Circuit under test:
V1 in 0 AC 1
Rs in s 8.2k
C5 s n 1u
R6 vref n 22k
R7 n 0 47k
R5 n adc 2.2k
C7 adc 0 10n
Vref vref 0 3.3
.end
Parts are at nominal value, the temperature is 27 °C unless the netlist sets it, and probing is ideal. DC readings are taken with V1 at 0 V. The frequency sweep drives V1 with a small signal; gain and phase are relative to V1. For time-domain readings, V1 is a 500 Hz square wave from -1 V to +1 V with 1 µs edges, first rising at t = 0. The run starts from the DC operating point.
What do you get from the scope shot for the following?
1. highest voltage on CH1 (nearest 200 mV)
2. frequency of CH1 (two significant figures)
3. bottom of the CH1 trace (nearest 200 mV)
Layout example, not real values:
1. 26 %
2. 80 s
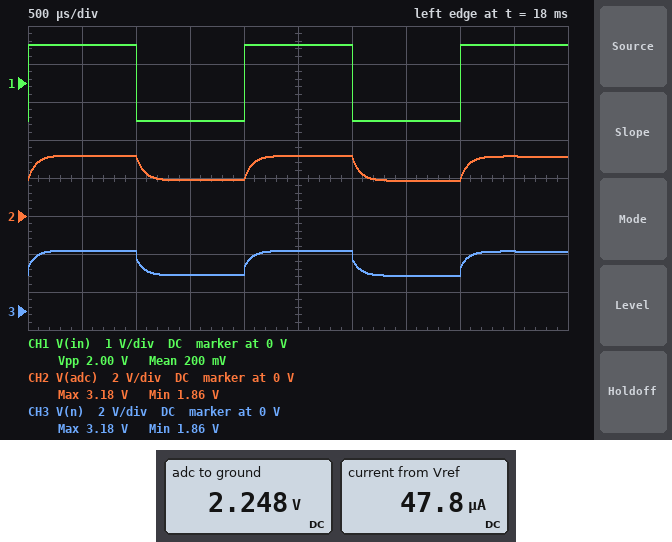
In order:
1. 1.0 V
2. 500 Hz
3. -1.0 V
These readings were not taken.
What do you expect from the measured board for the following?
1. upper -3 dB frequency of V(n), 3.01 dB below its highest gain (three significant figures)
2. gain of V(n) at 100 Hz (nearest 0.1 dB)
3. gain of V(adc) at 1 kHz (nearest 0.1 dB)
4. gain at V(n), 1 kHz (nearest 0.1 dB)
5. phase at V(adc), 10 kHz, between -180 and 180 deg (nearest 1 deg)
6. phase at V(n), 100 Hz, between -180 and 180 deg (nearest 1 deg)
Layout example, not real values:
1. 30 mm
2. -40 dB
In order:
1. 2.36 kHz
2. -3.9 dB
3. -4.7 dB
4. -4.6 dB
5. -78 deg
6. 2 deg
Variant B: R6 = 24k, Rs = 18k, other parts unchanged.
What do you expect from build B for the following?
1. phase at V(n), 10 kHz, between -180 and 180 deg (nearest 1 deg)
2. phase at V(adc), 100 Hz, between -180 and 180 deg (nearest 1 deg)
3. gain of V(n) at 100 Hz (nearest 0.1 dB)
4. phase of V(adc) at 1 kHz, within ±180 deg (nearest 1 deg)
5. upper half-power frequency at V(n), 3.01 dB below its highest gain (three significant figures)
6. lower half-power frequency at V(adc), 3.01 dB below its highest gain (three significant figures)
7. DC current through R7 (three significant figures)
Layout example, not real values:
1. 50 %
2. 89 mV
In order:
1. -27 deg
2. -1 deg
3. -6.6 dB
4. -33 deg
5. 1.58 kHz
6. 4.66 Hz
7. 46.5 µA
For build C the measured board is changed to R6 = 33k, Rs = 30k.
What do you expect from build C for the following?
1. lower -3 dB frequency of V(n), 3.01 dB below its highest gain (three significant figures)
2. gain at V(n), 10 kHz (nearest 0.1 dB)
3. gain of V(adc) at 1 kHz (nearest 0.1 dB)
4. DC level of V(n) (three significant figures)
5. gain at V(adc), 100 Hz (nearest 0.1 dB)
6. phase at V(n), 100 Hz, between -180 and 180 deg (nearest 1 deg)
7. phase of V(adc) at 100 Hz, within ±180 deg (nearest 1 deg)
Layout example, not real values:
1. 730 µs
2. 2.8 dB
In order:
1. 3.20 Hz
2. -22.4 dB
3. -10.6 dB
4. 1.94 V
5. -8.2 dB
6. -2 deg
7. -3 deg
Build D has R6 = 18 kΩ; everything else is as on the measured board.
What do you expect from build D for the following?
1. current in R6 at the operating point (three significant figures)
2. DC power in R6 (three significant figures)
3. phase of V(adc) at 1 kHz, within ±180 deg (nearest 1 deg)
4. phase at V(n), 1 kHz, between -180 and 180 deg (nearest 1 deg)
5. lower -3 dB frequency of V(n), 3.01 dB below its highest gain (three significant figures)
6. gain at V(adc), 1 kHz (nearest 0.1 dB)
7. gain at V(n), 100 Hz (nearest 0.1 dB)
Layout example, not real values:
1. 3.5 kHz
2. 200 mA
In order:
1. 50.8 µA
2. 46.4 µW
3. -24 deg
4. -16 deg
5. 7.43 Hz
6. -5.1 dB
7. -4.3 dB
